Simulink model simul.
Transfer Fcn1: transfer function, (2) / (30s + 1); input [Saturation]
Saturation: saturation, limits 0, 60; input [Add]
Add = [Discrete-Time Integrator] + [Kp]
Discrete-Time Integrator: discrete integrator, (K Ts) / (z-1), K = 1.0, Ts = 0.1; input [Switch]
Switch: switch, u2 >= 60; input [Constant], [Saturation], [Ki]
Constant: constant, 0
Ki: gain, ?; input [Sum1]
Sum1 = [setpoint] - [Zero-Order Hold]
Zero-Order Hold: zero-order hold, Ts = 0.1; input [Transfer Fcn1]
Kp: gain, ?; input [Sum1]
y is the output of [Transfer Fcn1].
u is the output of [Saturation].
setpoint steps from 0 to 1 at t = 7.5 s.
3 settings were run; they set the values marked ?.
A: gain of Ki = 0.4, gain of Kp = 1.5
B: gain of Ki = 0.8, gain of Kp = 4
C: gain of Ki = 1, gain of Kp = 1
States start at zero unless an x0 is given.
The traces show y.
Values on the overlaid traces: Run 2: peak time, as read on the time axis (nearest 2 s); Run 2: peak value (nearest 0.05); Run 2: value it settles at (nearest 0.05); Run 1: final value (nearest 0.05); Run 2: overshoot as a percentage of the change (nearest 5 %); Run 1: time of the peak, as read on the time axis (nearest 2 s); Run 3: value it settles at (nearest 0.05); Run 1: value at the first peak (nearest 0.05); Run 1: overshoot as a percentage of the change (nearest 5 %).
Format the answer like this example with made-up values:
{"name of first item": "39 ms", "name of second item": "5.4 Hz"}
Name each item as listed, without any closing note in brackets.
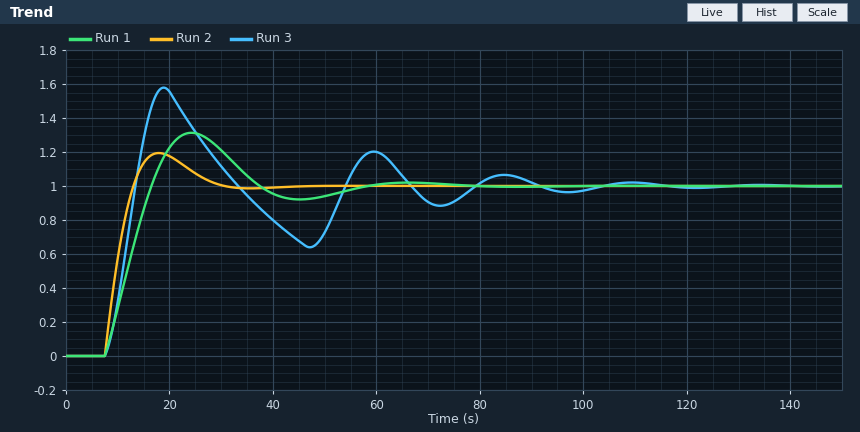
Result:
{"Run 2: peak time, as read on the time axis": "18 s", "Run 2: peak value": "1.20", "Run 2: value it settles at": "1.00", "Run 1: final value": "1.00", "Run 2: overshoot as a percentage of the change": "20 %", "Run 1: time of the peak, as read on the time axis": "24 s", "Run 3: value it settles at": "1.00", "Run 1: value at the first peak": "1.30", "Run 1: overshoot as a percentage of the change": "30 %"}
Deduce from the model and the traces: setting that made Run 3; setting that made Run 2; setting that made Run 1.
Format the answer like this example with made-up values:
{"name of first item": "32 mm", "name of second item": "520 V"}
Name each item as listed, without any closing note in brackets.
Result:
{"setting that made Run 3": "C", "setting that made Run 2": "B", "setting that made Run 1": "A"}
